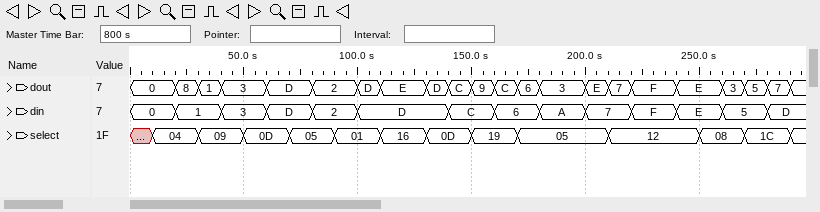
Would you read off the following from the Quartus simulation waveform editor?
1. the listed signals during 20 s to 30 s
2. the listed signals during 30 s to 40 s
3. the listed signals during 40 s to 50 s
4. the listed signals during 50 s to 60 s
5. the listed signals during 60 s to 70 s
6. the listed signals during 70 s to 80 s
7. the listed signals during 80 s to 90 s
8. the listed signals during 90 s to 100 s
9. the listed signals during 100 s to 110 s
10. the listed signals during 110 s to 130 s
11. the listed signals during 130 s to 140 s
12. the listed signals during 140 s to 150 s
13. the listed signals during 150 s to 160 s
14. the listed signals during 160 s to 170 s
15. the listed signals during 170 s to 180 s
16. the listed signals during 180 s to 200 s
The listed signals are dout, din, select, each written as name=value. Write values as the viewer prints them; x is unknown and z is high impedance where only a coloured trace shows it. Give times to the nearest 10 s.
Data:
dout=8, din=1, select=04
dout=1, din=1, select=09
dout=3, din=3, select=09
dout=3, din=3, select=0D
dout=D, din=D, select=0D
dout=D, din=D, select=05
dout=2, din=2, select=05
dout=2, din=2, select=01
dout=D, din=D, select=01
dout=E, din=D, select=16
dout=D, din=D, select=0D
dout=C, din=C, select=0D
dout=9, din=C, select=19
dout=C, din=6, select=19
dout=6, din=6, select=05
dout=3, din=A, select=05
